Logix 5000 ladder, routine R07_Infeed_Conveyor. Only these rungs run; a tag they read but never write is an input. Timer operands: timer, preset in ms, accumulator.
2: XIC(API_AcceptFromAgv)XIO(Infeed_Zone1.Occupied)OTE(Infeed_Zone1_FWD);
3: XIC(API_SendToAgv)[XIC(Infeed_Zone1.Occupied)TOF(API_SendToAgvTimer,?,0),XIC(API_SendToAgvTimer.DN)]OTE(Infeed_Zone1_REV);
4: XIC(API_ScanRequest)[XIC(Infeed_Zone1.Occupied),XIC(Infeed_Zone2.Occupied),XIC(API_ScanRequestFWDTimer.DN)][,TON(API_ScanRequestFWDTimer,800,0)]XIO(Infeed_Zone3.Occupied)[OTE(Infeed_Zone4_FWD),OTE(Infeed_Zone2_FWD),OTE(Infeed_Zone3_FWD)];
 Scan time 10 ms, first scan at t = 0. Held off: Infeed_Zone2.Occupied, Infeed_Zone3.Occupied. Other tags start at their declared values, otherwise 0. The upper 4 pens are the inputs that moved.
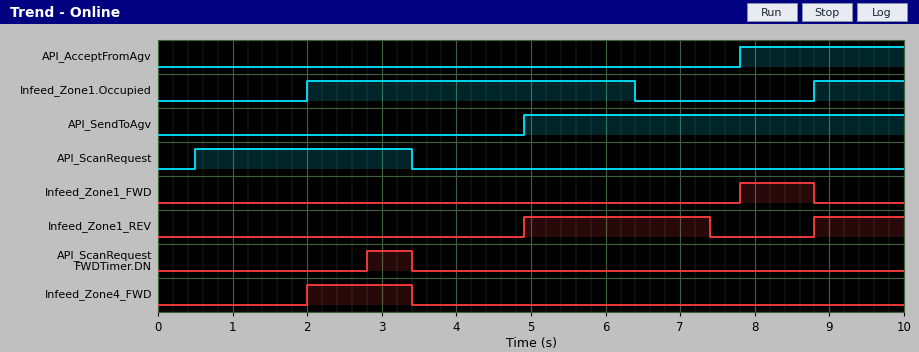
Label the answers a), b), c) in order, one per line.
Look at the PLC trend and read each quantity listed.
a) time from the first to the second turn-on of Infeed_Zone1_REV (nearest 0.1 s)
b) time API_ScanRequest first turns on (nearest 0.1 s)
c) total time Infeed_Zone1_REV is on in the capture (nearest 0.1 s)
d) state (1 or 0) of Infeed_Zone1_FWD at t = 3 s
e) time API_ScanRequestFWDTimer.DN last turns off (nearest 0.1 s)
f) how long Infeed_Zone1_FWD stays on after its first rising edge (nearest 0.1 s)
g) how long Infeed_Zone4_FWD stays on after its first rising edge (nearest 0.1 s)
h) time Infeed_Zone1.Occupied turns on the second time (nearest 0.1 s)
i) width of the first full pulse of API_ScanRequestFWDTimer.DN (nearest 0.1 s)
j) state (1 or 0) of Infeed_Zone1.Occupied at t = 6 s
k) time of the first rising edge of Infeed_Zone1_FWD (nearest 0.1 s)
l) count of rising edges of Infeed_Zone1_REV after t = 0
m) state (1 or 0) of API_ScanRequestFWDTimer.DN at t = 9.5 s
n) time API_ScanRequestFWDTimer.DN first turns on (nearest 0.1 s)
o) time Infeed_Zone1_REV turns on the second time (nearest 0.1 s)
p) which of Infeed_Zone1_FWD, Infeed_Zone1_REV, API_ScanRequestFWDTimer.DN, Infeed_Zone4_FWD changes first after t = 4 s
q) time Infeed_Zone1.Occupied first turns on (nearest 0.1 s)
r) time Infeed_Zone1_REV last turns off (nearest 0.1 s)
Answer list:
a) 3.9 s
b) 0.5 s
c) 3.7 s
d) 0
e) 3.4 s
f) 1.0 s
g) 1.4 s
h) 8.8 s
i) 0.6 s
j) 1
k) 7.8 s
l) 2
m) 0
n) 2.8 s
o) 8.8 s
p) Infeed_Zone1_REV
q) 2.0 s
r) 7.4 s
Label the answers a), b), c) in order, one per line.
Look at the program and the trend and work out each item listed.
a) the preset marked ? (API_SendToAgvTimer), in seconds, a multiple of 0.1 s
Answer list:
a) 1.0 s
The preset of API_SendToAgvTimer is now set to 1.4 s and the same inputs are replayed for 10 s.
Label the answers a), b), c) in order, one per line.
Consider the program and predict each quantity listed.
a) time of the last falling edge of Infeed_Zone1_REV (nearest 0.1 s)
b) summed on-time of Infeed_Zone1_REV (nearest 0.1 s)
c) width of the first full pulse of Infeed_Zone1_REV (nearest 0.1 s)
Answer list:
a) 7.8 s
b) 4.1 s
c) 2.9 s
